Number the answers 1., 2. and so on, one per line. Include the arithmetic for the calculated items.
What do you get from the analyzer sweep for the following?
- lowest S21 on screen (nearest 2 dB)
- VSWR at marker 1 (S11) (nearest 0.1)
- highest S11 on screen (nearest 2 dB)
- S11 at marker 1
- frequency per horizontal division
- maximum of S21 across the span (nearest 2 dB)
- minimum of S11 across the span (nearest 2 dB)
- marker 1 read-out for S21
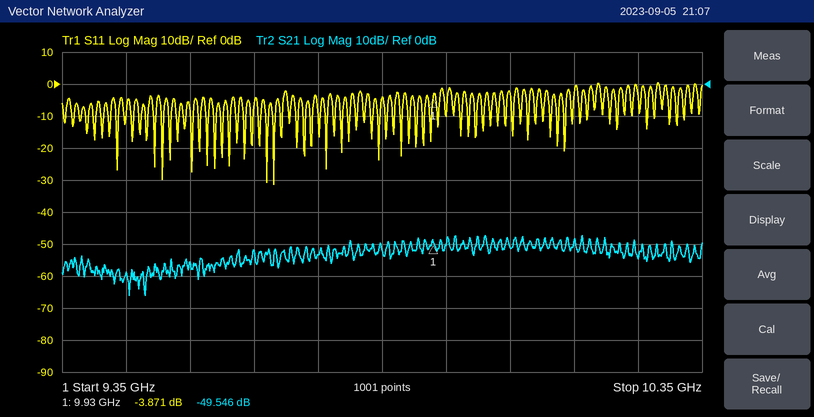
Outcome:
1. -66 dB
2. (1 + 0.6404)/(1 − 0.6404) ≈ 4.6
3. 0 dB
4. -3.871 dB
5. 100 MHz
6. -48 dB
7. -32 dB
8. -49.546 dB
